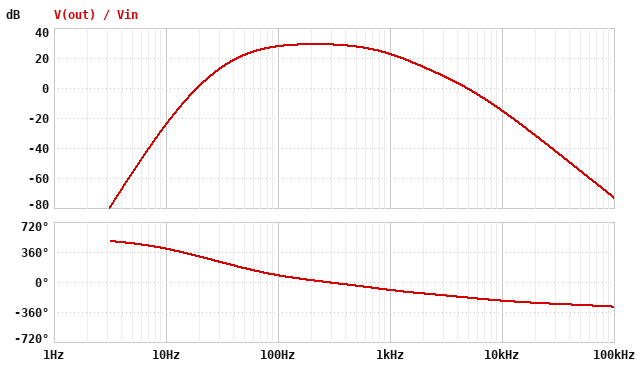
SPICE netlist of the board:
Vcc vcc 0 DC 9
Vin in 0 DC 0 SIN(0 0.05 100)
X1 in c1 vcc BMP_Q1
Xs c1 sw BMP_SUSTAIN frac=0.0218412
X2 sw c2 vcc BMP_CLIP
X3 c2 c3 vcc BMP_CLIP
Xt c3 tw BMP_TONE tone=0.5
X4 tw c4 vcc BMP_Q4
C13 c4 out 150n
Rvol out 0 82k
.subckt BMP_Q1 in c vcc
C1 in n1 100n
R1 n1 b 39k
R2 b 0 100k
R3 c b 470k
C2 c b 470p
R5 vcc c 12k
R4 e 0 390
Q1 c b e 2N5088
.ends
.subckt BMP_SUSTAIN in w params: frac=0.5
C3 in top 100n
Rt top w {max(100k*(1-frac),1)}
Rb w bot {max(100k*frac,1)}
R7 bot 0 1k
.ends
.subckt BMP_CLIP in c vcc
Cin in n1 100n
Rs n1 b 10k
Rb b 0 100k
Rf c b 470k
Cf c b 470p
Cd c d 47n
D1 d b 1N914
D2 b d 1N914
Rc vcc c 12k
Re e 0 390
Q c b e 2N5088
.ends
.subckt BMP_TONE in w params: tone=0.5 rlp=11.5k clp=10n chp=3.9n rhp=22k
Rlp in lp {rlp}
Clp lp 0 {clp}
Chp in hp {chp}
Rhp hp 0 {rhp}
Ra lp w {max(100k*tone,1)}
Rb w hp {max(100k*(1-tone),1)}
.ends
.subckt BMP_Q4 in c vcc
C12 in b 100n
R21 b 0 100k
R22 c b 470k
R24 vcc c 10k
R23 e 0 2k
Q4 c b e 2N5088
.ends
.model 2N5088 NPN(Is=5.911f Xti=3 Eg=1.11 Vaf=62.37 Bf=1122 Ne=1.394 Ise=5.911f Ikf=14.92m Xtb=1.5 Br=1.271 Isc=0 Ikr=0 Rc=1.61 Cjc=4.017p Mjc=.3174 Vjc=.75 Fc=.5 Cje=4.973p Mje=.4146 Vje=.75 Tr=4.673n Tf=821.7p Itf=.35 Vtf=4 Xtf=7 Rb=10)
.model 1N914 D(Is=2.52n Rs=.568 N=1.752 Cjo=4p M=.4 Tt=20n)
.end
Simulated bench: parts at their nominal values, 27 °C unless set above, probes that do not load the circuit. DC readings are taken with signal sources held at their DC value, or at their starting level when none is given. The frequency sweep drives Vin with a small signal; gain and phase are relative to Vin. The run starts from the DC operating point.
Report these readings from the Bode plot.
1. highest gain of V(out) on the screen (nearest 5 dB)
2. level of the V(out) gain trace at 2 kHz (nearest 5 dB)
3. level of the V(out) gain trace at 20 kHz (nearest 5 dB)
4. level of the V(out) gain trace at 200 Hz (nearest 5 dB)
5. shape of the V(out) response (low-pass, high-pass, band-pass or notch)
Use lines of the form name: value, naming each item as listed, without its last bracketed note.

highest gain of V(out) on the screen: 30 dB
level of the V(out) gain trace at 2 kHz: 15 dB
level of the V(out) gain trace at 20 kHz: -30 dB
level of the V(out) gain trace at 200 Hz: 30 dB
shape of the V(out) response: band-pass
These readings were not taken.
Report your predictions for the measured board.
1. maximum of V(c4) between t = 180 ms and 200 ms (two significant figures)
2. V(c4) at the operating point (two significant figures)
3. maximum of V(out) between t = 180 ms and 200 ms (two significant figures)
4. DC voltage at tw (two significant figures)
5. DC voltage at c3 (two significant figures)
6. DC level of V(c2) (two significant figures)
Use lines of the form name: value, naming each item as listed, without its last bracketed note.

maximum of V(c4) between t = 180 ms and 200 ms: 6.9 V
V(c4) at the operating point: 6.5 V
maximum of V(out) between t = 180 ms and 200 ms: 410 mV
DC voltage at tw: 2.5 V
DC voltage at c3: 4.6 V
DC level of V(c2): 4.7 V
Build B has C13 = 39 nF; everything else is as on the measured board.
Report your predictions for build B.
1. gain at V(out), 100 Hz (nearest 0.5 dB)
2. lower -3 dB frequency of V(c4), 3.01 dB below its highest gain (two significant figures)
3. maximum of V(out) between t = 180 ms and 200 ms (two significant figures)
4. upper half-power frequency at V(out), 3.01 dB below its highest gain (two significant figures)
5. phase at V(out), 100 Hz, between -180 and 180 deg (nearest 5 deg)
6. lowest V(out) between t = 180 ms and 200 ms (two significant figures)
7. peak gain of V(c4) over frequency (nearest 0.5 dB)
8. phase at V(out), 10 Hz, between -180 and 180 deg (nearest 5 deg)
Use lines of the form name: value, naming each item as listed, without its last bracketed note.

gain at V(out), 100 Hz: 27.0 dB
lower -3 dB frequency of V(c4), 3.01 dB below its highest gain: 72 Hz
maximum of V(out) between t = 180 ms and 200 ms: 440 mV
upper half-power frequency at V(out), 3.01 dB below its highest gain: 670 Hz
phase at V(out), 100 Hz, between -180 and 180 deg: 100 deg
lowest V(out) between t = 180 ms and 200 ms: -440 mV
peak gain of V(c4) over frequency: 29.5 dB
phase at V(out), 10 Hz, between -180 and 180 deg: 70 deg
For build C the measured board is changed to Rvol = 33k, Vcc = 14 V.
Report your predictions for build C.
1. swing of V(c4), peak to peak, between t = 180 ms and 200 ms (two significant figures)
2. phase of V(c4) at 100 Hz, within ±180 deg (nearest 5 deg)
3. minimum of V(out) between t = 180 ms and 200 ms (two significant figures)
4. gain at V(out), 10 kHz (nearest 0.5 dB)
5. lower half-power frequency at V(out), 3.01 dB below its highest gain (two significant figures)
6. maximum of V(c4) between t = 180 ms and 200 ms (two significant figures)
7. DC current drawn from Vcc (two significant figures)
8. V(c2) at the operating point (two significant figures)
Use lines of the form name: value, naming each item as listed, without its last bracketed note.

swing of V(c4), peak to peak, between t = 180 ms and 200 ms: 820 mV
phase of V(c4) at 100 Hz, within ±180 deg: 75 deg
minimum of V(out) between t = 180 ms and 200 ms: -380 mV
gain at V(out), 10 kHz: -15.5 dB
lower half-power frequency at V(out), 3.01 dB below its highest gain: 80 Hz
maximum of V(c4) between t = 180 ms and 200 ms: 9.7 V
DC current drawn from Vcc: 2.5 mA
V(c2) at the operating point: 5.8 V
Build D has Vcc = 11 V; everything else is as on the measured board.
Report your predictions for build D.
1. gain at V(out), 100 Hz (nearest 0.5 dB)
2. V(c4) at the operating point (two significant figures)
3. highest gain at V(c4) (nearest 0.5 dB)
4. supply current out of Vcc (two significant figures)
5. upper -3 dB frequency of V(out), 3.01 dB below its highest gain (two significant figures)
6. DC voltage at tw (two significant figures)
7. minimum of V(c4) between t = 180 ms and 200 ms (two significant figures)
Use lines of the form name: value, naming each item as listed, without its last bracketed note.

gain at V(out), 100 Hz: 28.5 dB
V(c4) at the operating point: 7.6 V
highest gain at V(c4): 30.0 dB
supply current out of Vcc: 1.8 mA
upper -3 dB frequency of V(out), 3.01 dB below its highest gain: 650 Hz
DC voltage at tw: 2.7 V
minimum of V(c4) between t = 180 ms and 200 ms: 7.2 V
